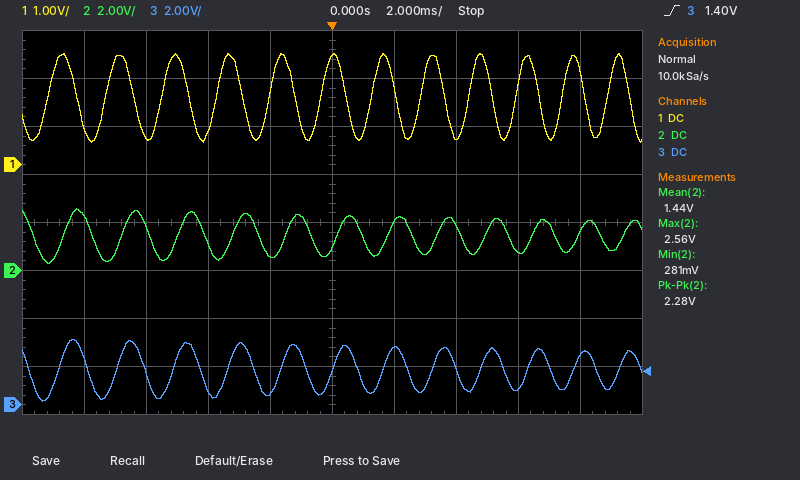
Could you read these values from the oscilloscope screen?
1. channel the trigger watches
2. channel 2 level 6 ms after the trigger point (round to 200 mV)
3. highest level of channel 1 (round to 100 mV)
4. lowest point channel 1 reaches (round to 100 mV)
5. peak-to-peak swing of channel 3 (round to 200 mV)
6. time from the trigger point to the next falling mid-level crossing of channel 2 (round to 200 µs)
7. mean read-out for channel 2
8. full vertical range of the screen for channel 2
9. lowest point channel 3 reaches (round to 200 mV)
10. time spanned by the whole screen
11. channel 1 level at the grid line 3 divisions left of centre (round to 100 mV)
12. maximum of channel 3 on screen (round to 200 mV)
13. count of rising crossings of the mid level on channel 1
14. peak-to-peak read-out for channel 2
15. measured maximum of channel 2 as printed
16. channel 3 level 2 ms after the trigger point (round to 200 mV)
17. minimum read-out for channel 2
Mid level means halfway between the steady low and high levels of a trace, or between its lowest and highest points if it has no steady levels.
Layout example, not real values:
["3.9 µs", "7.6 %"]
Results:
["channel 3", "800 mV", "2.3 V", "500 mV", "2.6 V", "1.0 ms", "1.44 V", "16 V", "200 mV", "20 ms", "600 mV", "2.8 V", "12", "2.28 V", "2.56 V", "2.4 V", "281 mV"]
